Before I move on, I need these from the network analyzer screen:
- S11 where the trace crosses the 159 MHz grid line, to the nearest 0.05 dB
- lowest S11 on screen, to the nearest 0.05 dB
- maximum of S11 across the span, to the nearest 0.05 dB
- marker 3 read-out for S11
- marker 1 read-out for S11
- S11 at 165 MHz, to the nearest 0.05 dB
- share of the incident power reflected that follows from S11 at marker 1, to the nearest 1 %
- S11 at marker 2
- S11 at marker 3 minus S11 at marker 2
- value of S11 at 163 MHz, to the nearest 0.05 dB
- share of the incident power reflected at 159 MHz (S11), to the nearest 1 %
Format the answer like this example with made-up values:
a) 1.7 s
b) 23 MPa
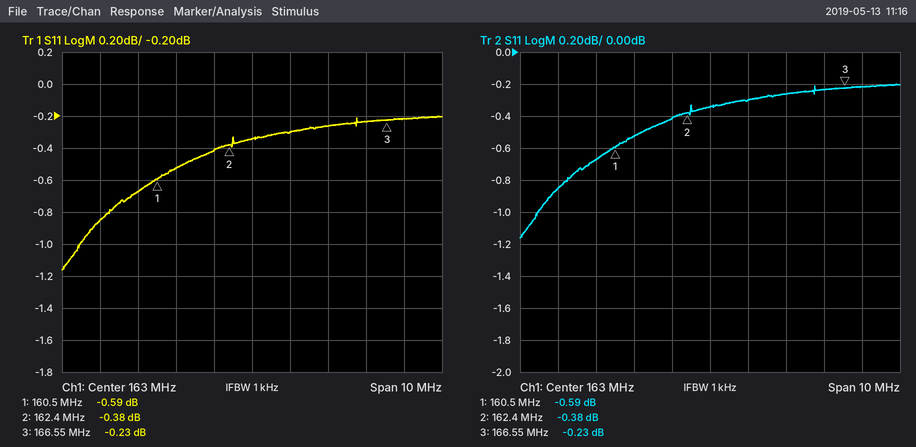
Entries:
a) -0.85 dB
b) -1.15 dB
c) -0.20 dB
d) -0.23 dB
e) -0.59 dB
f) -0.25 dB
g) 87 %
h) -0.38 dB
i) 0.15 dB
j) -0.35 dB
k) 82 %
